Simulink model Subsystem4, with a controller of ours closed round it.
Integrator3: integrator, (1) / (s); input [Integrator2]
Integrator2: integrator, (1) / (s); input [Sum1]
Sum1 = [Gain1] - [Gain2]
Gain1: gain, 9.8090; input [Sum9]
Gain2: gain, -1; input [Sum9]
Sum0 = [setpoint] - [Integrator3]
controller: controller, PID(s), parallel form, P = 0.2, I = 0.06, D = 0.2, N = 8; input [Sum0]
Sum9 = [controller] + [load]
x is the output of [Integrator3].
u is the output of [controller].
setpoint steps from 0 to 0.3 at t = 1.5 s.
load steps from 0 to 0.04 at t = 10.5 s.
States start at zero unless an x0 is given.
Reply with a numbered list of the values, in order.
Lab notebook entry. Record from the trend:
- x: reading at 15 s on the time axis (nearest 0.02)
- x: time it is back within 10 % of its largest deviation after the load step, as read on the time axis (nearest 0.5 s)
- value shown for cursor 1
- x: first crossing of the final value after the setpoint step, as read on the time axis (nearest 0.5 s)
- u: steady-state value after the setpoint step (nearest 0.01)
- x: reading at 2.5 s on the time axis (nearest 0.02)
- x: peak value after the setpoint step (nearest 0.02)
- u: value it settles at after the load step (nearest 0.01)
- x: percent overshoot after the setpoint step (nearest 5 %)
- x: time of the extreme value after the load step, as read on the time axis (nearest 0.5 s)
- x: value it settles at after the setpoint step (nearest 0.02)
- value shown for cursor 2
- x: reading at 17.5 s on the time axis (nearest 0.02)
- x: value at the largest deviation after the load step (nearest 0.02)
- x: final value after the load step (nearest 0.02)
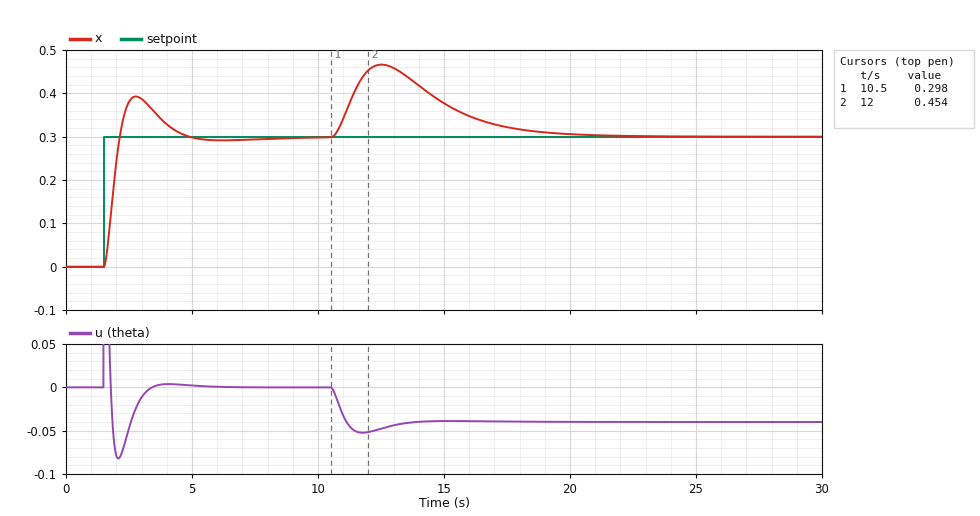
1. 0.38
2. 18.0 s
3. 0.298
4. 2.0 s
5. 0.00
6. 0.38
7. 0.40
8. -0.04
9. 30 %
10. 12.5 s
11. 0.30
12. 0.454
13. 0.32
14. 0.46
15. 0.30
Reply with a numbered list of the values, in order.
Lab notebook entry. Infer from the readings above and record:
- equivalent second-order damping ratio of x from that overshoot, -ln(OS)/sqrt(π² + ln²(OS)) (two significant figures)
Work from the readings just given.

1. 0.36
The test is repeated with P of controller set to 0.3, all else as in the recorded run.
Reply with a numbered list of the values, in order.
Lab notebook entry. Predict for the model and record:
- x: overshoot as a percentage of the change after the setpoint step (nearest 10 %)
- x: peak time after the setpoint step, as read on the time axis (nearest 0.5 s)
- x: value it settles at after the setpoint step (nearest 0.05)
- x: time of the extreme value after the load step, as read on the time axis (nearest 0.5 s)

1. 40 %
2. 2.5 s
3. 0.30
4. 12.0 s
